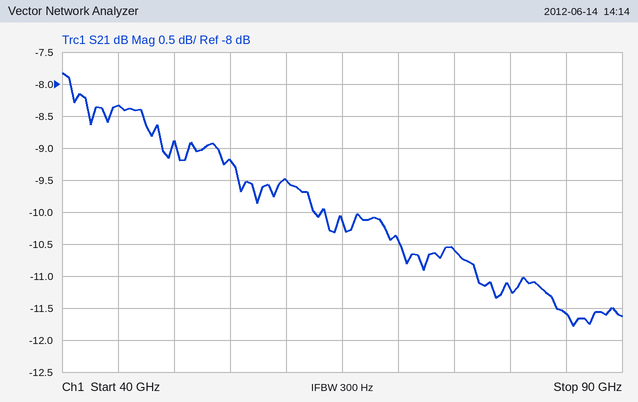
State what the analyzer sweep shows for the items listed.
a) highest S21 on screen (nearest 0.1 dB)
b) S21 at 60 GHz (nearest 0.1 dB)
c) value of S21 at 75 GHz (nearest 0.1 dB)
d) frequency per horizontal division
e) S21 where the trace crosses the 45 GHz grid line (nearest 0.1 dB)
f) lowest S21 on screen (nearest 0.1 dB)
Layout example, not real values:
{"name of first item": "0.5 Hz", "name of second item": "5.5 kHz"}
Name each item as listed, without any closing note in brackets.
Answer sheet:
{"highest S21 on screen": "-7.8 dB", "S21 at 60 GHz": "-9.5 dB", "value of S21 at 75 GHz": "-10.6 dB", "frequency per horizontal division": "5 GHz", "S21 where the trace crosses the 45 GHz grid line": "-8.3 dB", "lowest S21 on screen": "-11.8 dB"}
